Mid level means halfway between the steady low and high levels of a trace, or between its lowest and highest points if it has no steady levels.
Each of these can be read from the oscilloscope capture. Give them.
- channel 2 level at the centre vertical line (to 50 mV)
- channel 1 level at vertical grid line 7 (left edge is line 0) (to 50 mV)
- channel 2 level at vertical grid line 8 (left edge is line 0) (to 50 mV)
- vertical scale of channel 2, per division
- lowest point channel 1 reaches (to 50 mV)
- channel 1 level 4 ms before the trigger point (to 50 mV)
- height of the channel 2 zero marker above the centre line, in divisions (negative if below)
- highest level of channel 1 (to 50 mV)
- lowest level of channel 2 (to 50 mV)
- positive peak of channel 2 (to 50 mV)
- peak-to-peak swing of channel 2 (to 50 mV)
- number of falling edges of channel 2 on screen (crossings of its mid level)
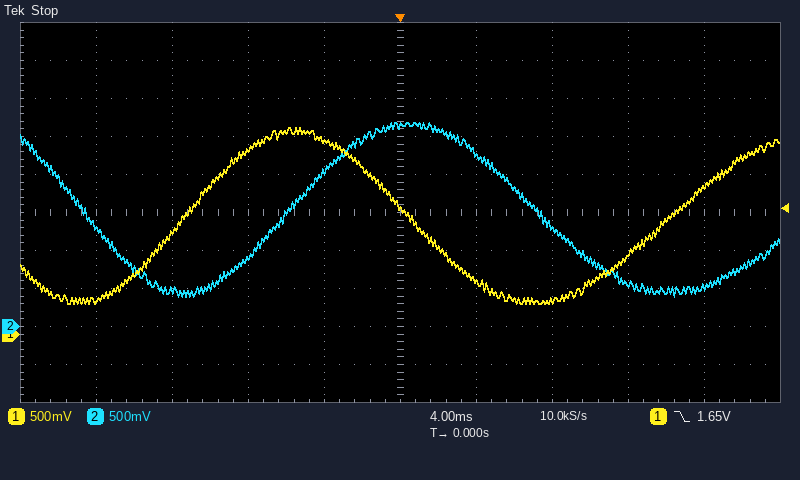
2.65 V
450 mV
550 mV
500 mV
400 mV
2.55 V
-3.0 div
2.70 V
400 mV
2.70 V
2.30 V
2
